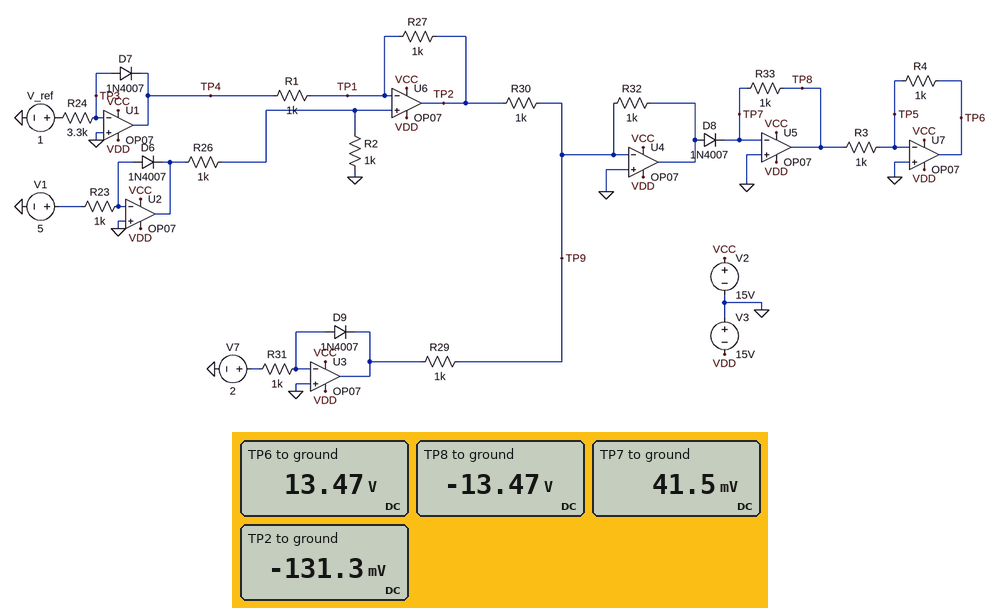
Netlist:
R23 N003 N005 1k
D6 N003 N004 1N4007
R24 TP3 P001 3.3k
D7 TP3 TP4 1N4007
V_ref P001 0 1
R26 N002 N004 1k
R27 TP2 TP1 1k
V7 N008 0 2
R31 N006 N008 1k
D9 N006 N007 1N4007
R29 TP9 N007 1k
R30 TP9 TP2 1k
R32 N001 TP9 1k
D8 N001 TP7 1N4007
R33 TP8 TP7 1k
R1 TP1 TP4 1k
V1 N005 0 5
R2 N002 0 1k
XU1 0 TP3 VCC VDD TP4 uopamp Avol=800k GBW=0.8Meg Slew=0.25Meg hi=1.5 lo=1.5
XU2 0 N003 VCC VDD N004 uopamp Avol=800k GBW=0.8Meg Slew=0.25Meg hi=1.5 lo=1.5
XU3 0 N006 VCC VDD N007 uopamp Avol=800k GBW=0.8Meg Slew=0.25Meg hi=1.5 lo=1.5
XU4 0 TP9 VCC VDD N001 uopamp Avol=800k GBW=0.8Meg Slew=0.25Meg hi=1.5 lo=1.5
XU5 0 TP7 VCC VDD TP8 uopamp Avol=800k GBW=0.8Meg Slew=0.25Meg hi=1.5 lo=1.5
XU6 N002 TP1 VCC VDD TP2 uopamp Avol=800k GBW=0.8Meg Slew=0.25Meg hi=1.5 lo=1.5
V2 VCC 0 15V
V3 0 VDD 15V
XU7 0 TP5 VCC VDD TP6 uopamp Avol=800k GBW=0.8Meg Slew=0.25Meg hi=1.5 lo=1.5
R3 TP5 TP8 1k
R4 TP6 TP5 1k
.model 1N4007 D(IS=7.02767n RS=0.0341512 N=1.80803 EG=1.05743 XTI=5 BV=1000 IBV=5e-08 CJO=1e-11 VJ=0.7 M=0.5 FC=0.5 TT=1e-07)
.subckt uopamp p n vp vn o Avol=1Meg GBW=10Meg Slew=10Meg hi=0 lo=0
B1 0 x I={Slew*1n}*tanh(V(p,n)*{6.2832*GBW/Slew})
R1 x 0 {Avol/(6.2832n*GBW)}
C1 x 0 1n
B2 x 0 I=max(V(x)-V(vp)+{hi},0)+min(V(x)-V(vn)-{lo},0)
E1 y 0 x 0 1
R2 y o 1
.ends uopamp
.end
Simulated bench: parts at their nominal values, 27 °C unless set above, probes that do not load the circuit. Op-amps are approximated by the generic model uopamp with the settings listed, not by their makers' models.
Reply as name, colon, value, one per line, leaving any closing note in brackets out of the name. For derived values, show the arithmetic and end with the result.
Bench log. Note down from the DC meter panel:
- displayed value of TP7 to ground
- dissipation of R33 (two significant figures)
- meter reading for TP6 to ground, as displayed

displayed value of TP7 to ground: 41.5 mV
dissipation of R33: (41.5 mV - (-13.47 V))^2 / 1 kΩ = 180 mW
meter reading for TP6 to ground, as displayed: 13.47 V
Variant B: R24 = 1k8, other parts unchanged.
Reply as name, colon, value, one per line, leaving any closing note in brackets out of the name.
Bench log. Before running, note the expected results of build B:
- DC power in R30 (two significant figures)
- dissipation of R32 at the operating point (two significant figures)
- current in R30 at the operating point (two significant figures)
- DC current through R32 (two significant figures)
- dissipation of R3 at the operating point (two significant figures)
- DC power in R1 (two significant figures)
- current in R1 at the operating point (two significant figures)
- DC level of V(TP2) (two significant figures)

DC power in R30: 11 µW
dissipation of R32 at the operating point: 480 µW
current in R30 at the operating point: 100 µA
DC current through R32: 690 µA
dissipation of R3 at the operating point: 180 mW
DC power in R1: 45 µW
current in R1 at the operating point: 210 µA
DC level of V(TP2): -100 mV
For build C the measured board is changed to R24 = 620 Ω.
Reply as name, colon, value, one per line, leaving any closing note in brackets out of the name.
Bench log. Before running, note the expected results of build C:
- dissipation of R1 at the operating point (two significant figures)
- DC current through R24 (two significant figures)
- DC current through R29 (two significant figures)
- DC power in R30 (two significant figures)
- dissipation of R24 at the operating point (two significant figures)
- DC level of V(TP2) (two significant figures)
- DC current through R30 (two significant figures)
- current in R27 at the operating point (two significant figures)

dissipation of R1 at the operating point: 69 µW
DC current through R24: 1.6 mA
DC current through R29: 590 µA
DC power in R30: 2.8 µW
dissipation of R24 at the operating point: 1.6 mW
DC level of V(TP2): -53 mV
DC current through R30: 53 µA
current in R27 at the operating point: 260 µA
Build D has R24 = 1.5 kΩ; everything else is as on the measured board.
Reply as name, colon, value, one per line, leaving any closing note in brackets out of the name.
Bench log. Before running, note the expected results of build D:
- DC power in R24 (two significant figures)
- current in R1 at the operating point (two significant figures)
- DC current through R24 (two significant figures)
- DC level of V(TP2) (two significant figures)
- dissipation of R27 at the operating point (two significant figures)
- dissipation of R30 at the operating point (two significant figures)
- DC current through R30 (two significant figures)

DC power in R24: 670 µW
current in R1 at the operating point: 220 µA
DC current through R24: 670 µA
DC level of V(TP2): -94 mV
dissipation of R27 at the operating point: 49 µW
dissipation of R30 at the operating point: 8.9 µW
DC current through R30: 94 µA
